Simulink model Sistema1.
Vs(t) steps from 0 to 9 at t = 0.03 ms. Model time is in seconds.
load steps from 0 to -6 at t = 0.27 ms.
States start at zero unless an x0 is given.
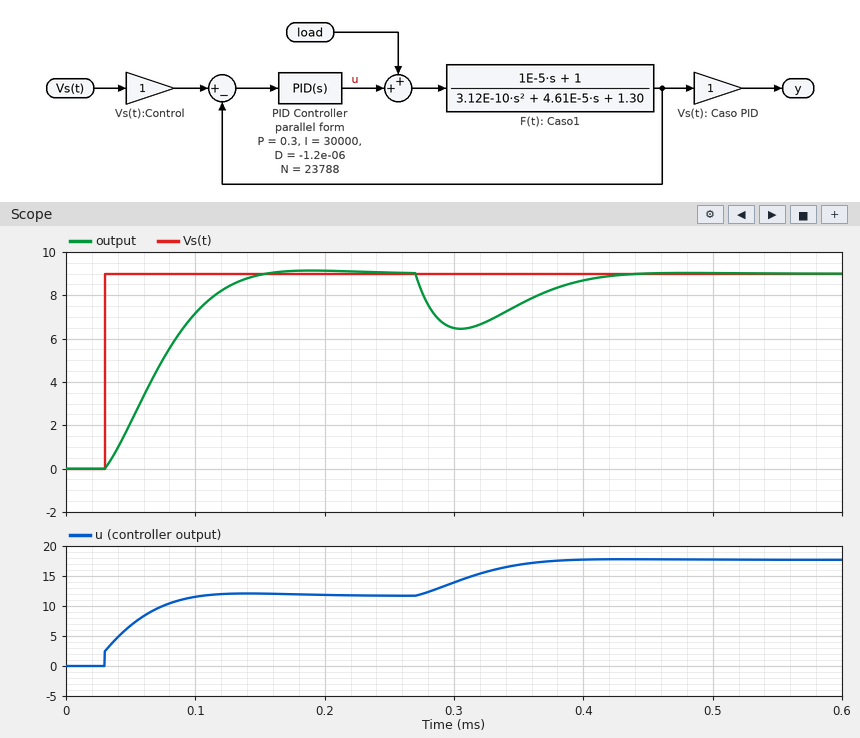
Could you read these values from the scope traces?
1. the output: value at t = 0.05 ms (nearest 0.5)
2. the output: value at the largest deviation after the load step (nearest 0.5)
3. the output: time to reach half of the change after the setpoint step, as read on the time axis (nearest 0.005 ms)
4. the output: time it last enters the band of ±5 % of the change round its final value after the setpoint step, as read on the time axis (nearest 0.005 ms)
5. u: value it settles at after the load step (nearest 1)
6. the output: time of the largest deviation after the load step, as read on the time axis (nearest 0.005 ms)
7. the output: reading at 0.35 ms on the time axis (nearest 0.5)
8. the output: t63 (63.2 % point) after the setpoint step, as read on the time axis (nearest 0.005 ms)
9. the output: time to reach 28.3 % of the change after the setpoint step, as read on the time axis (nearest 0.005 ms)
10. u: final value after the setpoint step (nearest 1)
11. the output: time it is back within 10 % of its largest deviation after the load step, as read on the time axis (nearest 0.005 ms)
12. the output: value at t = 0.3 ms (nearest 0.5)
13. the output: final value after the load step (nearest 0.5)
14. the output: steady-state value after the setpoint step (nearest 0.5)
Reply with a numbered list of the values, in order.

1. 2.0
2. 6.5
3. 0.070 ms
4. 0.130 ms
5. 18
6. 0.305 ms
7. 7.5
8. 0.080 ms
9. 0.055 ms
10. 12
11. 0.405 ms
12. 6.5
13. 9.0
14. 9.0
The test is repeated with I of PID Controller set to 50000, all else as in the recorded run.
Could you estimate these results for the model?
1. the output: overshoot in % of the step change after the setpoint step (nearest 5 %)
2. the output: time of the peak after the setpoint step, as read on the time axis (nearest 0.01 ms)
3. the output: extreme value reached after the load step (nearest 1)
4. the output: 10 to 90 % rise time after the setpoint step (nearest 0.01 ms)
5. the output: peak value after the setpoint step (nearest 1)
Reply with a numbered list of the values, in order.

1. 10 %
2. 0.13 ms
3. 7
4. 0.05 ms
5. 10
